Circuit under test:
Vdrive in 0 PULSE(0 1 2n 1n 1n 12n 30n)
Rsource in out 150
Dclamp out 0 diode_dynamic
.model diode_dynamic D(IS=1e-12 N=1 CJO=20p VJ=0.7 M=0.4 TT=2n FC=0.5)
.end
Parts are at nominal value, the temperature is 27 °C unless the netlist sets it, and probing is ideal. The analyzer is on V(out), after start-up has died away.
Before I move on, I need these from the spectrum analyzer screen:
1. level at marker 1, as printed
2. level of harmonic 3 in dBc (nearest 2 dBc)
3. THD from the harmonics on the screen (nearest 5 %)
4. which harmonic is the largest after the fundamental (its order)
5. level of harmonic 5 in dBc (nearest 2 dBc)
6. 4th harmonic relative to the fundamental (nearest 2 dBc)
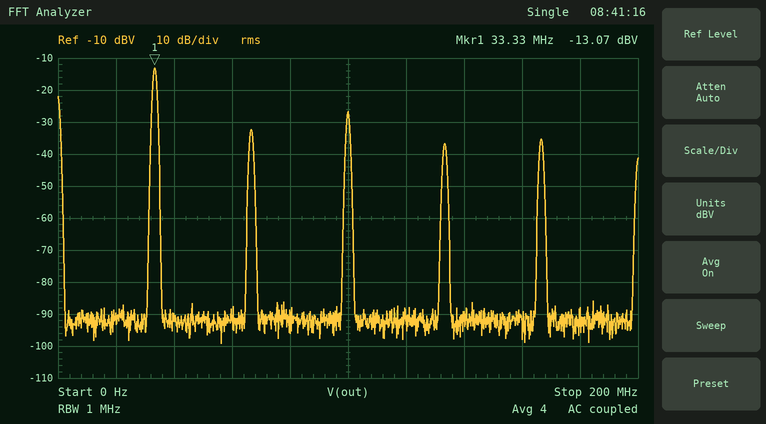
-13.07 dBV
-14 dBc
25 %
3
-22 dBc
-24 dBc
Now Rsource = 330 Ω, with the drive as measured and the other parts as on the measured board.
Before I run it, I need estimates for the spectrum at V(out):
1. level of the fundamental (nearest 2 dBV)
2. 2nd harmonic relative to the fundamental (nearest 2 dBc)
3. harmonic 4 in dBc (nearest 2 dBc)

-16 dBV
-16 dBc
-26 dBc
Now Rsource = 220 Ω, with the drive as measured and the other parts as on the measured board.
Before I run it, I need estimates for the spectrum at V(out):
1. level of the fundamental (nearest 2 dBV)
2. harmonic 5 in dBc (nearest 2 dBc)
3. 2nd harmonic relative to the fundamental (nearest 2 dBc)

-14 dBV
-26 dBc
-16 dBc
